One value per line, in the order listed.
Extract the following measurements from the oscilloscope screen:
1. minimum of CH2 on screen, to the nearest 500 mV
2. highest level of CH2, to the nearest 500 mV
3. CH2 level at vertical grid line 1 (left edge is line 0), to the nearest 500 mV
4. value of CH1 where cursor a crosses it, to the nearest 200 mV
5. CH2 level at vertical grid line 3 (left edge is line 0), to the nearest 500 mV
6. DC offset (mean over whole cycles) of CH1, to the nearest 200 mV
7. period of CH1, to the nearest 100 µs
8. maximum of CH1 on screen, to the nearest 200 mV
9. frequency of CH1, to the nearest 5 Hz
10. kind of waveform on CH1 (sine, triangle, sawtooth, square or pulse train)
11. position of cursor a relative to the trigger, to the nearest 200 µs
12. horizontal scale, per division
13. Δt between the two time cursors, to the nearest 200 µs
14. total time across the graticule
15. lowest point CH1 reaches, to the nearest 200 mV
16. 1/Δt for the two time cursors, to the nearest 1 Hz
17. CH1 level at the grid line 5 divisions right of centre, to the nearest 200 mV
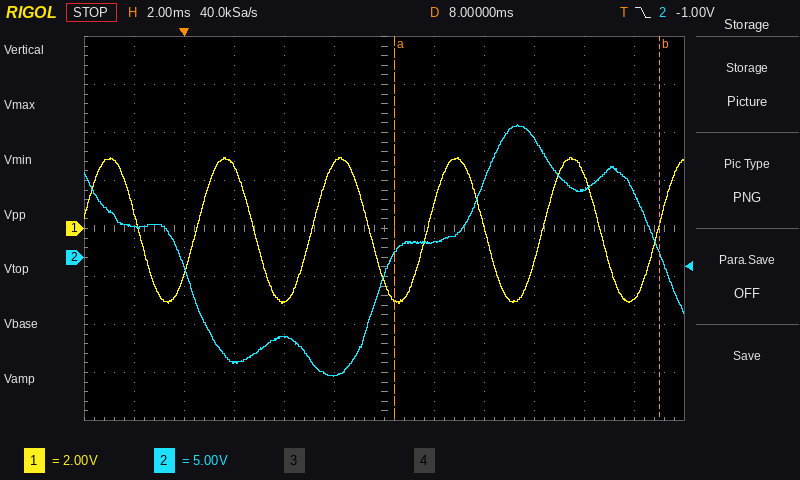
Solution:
-12.5 V
14.0 V
3.0 V
-3.0 V
-11.0 V
0.0 V
4.6 ms
3.0 V
215 Hz
sine
+8.4 ms
2 ms
10.6 ms
24 ms
-3.2 V
94 Hz
-3.0 V
